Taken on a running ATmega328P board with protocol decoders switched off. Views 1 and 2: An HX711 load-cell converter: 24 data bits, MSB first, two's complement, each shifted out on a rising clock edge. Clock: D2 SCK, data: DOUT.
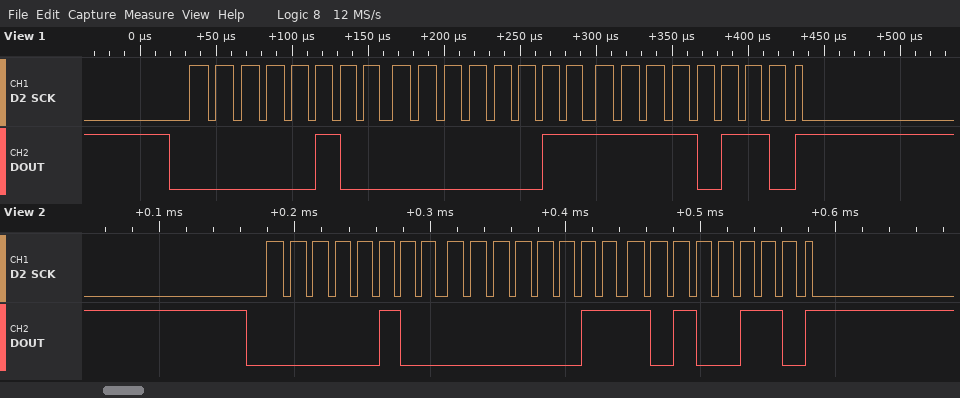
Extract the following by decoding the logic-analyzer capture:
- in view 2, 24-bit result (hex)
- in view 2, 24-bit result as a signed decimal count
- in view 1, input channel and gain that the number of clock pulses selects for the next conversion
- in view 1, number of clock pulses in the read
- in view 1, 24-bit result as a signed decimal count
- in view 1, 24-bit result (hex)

0x0403A6
263078
channel A, gain 128
25
263158
0x0403F6
